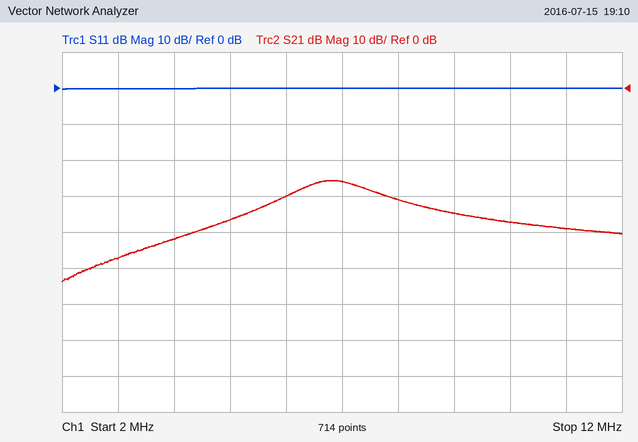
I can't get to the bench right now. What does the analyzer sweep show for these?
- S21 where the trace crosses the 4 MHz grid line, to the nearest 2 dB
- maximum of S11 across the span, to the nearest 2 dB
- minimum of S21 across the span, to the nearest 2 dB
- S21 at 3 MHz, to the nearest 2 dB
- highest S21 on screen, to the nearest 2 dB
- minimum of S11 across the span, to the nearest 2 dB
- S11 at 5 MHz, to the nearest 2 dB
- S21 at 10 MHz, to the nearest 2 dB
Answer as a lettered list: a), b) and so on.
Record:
a) -42 dB
b) 0 dB
c) -54 dB
d) -48 dB
e) -26 dB
f) 0 dB
g) 0 dB
h) -38 dB
